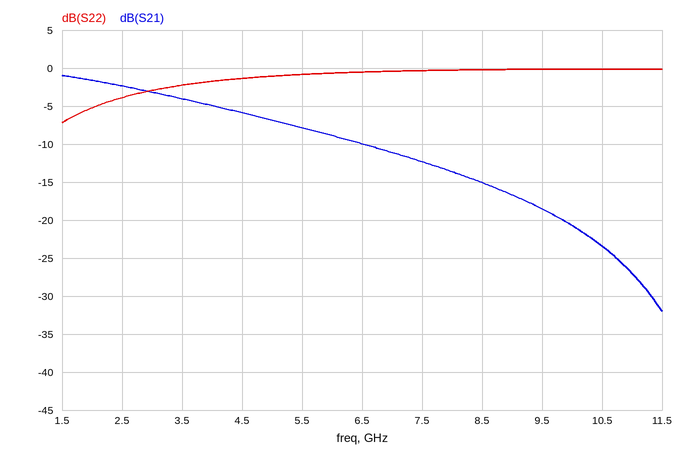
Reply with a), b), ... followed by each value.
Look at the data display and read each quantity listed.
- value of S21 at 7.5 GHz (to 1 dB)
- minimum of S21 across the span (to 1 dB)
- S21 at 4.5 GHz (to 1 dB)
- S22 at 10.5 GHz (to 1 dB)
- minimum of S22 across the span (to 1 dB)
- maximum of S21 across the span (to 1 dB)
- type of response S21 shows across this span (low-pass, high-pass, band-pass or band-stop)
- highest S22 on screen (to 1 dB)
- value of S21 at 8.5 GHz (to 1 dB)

a) -12 dB
b) -32 dB
c) -6 dB
d) 0 dB
e) -7 dB
f) -1 dB
g) low-pass
h) 0 dB
i) -15 dB
